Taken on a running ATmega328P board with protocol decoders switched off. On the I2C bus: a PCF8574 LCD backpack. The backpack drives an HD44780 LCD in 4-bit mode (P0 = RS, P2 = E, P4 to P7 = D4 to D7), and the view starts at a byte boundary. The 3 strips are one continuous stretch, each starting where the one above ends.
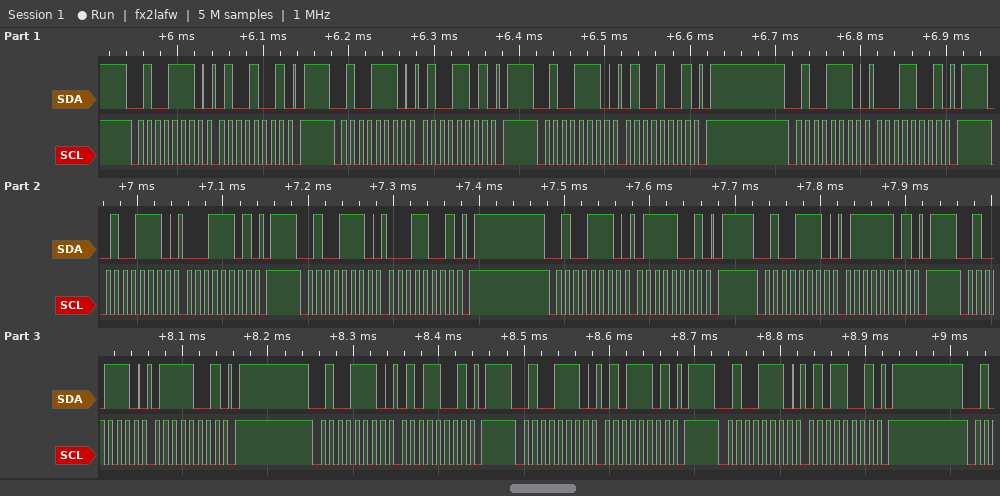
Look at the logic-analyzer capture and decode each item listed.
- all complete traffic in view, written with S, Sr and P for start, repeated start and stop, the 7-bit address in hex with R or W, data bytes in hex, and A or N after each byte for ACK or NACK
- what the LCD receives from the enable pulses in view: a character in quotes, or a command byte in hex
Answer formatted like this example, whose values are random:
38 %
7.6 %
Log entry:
S 27W A 49 A P S 27W A 4D A P S 27W A 49 A P S 27W A 19 A P S 27W A 1D A P S 27W A 19 A P S 27W A 79 A P S 27W A 7D A P S 27W A 79 A P S 27W A 59 A P S 27W A 5D A P S 27W A 59 A P
'A' 'u'
